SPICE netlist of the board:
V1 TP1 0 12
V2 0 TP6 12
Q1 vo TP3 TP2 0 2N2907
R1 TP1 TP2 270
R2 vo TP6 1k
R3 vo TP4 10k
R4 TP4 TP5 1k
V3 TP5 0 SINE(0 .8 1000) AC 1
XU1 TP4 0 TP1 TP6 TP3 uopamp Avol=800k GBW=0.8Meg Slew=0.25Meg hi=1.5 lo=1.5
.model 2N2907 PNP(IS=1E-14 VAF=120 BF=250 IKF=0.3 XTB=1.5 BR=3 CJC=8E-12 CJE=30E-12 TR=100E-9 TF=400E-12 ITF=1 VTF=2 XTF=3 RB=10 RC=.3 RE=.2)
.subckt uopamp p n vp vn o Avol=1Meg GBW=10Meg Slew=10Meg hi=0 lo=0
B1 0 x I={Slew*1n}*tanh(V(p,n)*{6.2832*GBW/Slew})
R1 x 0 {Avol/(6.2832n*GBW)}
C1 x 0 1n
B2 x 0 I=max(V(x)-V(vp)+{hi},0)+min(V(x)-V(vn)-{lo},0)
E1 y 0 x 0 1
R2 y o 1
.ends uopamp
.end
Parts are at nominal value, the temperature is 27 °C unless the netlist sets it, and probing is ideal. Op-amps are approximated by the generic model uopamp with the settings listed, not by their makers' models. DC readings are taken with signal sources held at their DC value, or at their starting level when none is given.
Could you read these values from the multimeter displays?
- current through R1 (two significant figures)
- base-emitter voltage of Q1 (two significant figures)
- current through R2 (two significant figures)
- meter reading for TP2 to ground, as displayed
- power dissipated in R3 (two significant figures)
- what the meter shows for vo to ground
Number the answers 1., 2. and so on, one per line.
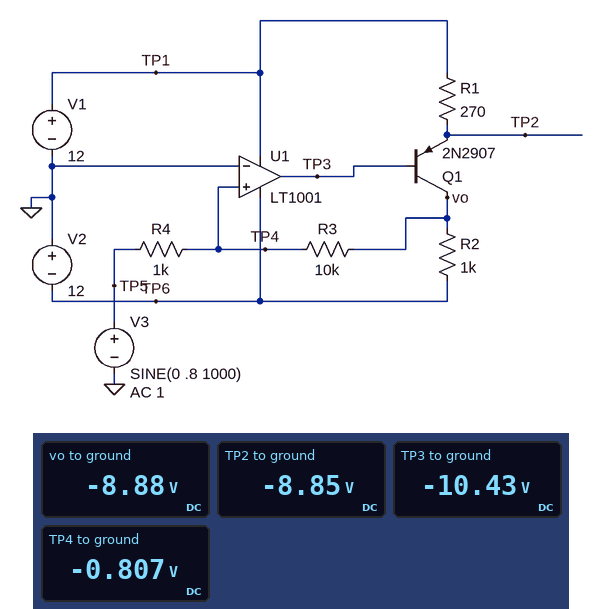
1. 77 mA
2. -1.6 V
3. 3.1 mA
4. -8.85 V
5. 6.5 mW
6. -8.88 V
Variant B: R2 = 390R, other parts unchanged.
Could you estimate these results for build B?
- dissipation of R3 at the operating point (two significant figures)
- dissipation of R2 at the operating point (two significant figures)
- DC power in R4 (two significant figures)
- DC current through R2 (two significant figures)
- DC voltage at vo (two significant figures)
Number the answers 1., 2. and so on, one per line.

1. 6.6 mW
2. 24 mW
3. 660 µW
4. 7.9 mA
5. -8.9 V
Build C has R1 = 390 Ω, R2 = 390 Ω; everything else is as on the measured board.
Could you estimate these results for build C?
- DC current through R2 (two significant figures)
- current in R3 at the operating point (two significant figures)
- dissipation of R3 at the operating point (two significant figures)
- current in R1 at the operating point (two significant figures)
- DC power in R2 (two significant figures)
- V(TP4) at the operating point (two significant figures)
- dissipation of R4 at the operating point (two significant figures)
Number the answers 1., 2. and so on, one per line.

1. 7.2 mA
2. 840 µA
3. 7.0 mW
4. 54 mA
5. 20 mW
6. -840 mV
7. 700 µW
